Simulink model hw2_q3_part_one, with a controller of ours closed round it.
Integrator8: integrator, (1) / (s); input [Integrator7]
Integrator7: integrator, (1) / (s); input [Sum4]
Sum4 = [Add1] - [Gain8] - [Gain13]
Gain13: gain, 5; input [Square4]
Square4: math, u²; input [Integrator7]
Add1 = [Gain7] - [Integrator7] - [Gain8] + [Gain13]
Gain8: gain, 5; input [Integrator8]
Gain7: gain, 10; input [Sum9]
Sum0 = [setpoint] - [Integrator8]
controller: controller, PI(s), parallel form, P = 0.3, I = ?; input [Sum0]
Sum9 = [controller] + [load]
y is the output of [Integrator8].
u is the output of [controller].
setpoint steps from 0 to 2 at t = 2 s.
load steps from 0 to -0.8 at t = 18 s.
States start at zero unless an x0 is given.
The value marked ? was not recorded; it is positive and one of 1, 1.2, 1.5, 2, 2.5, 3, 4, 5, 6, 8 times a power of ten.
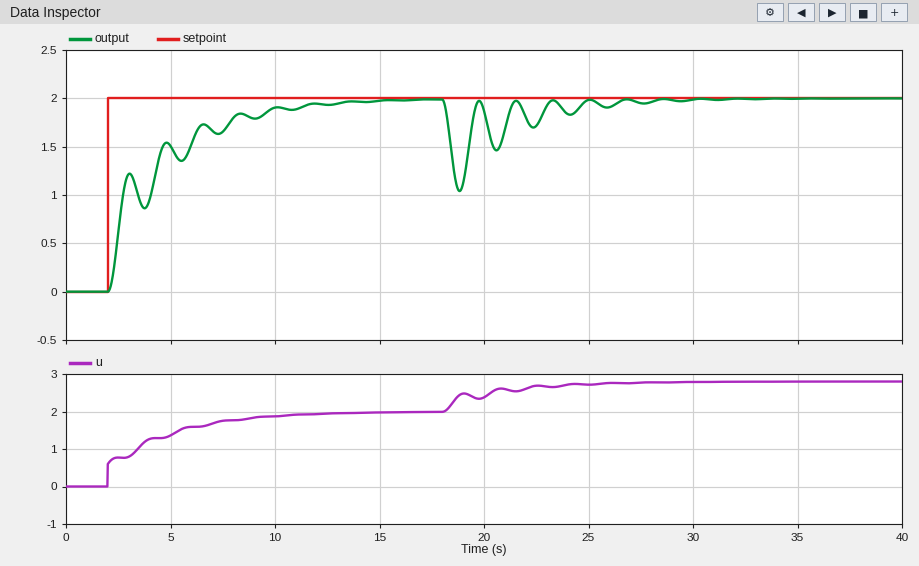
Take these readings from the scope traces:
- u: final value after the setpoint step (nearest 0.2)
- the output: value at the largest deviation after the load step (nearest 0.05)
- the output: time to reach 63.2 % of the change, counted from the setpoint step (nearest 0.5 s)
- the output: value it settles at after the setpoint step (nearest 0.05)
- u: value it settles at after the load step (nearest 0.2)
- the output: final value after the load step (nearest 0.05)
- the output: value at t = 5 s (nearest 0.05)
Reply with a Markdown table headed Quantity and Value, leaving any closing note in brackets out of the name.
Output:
| Quantity | Value |
|---|---|
| u: final value after the setpoint step | 2.0 |
| the output: value at the largest deviation after the load step | 1.05 |
| the output: time to reach 63.2 % of the change, counted from the setpoint step | 2.5 s |
| the output: value it settles at after the setpoint step | 2.00 |
| u: value it settles at after the load step | 2.8 |
| the output: final value after the load step | 2.00 |
| the output: value at t = 5 s | 1.50 |
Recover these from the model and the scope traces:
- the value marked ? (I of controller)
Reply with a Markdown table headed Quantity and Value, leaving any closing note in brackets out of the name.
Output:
| Quantity | Value |
|---|---|
| the value marked ? | 0.4 |
